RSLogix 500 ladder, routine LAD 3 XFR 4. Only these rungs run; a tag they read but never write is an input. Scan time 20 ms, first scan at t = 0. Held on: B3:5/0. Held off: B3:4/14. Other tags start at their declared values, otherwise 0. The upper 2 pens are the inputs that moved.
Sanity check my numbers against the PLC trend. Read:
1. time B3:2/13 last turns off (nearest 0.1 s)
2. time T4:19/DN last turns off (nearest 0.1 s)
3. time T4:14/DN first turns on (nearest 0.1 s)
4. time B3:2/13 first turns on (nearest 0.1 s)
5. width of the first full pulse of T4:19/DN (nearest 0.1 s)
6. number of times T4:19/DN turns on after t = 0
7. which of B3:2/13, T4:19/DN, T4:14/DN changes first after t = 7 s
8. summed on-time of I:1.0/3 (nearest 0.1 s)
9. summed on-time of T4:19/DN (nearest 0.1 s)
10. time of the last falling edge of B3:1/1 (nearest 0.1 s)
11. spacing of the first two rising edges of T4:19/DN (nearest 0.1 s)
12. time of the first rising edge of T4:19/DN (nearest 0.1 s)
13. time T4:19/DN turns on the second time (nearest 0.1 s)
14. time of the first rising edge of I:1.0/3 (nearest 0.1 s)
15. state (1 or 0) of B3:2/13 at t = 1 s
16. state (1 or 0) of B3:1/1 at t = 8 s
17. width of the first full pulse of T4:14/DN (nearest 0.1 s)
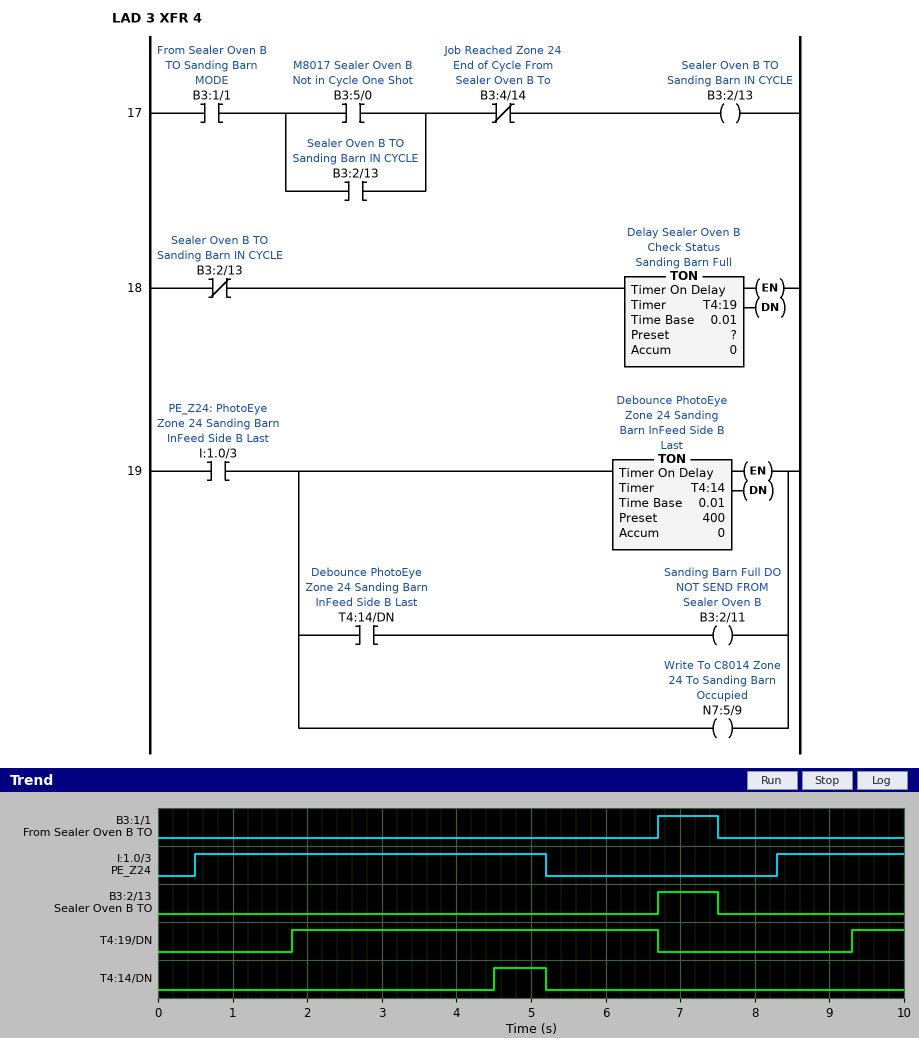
7.5 s
6.7 s
4.5 s
6.7 s
4.9 s
2
B3:2/13
6.4 s
5.6 s
7.5 s
7.5 s
1.8 s
9.3 s
0.5 s
0
0
0.7 s
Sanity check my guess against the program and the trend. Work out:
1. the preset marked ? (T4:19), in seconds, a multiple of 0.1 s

1.8 s
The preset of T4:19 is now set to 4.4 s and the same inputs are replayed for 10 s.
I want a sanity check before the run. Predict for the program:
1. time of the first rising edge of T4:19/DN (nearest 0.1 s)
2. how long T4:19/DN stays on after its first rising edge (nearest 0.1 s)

4.4 s
2.3 s
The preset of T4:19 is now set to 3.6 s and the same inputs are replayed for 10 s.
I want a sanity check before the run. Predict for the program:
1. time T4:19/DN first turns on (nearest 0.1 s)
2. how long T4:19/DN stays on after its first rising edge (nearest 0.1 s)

3.6 s
3.1 s
